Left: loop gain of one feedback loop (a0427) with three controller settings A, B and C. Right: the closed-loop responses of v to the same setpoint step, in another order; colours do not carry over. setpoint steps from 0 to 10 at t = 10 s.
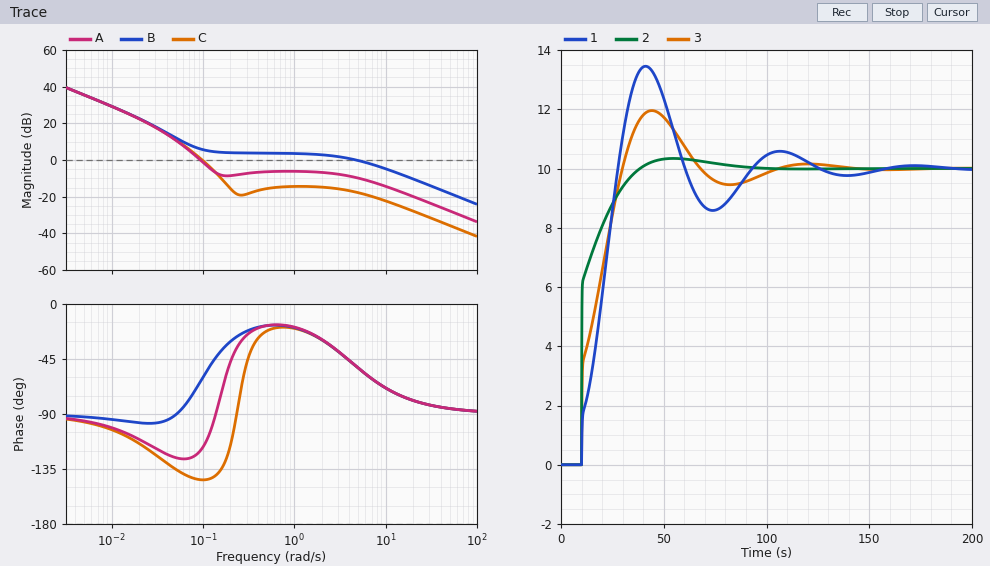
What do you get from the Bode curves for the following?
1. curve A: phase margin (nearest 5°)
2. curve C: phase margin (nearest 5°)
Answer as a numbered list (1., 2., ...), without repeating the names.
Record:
1. 60°
2. 35°
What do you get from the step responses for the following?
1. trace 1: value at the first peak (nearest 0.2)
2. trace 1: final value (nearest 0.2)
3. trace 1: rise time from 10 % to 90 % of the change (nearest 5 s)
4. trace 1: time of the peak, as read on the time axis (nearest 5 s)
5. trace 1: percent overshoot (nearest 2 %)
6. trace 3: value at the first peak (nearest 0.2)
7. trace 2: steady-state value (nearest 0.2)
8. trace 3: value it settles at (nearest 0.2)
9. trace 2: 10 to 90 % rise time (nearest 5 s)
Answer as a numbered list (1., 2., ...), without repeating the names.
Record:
1. 13.4
2. 10.0
3. 15 s
4. 40 s
5. 34 %
6. 12.0
7. 10.0
8. 10.0
9. 15 s
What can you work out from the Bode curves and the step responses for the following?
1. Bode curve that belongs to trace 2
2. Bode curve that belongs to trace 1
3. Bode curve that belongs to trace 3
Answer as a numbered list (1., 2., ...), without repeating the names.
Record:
1. B
2. C
3. A
